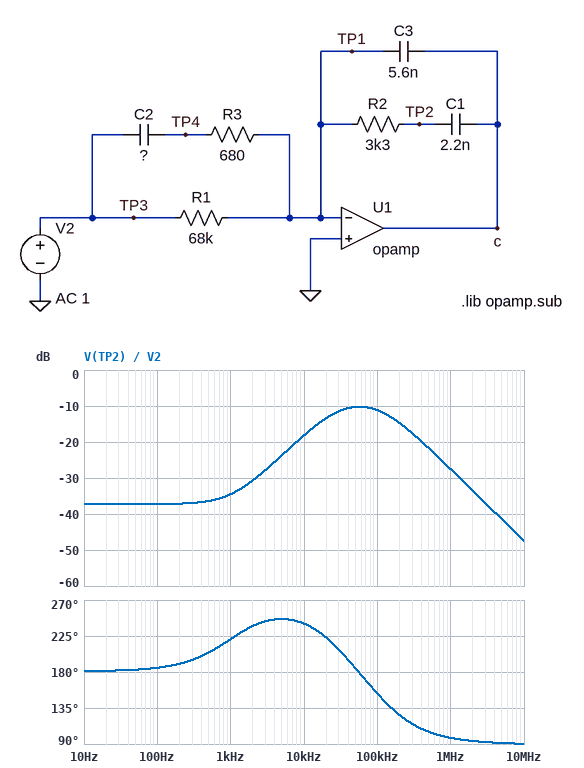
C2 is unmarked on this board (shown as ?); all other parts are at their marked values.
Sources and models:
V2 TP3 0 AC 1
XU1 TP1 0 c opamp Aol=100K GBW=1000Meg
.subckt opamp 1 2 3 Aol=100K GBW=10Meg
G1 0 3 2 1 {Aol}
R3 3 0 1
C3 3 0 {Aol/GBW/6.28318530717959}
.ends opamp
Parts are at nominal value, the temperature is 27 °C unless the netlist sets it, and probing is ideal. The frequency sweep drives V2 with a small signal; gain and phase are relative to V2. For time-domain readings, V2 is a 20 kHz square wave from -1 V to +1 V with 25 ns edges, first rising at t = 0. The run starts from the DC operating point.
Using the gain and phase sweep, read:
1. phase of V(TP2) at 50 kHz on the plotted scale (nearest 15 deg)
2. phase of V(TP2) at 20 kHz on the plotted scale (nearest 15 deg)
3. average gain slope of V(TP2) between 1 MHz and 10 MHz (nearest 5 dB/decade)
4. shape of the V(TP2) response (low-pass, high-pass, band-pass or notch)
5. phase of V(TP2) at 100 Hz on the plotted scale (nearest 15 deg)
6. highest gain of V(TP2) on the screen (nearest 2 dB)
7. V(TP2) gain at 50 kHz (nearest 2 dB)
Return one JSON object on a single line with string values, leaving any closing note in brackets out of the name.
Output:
{"phase of V(TP2) at 50 kHz on the plotted scale": "180 deg", "phase of V(TP2) at 20 kHz on the plotted scale": "225 deg", "average gain slope of V(TP2) between 1 MHz and 10 MHz": "-20 dB/decade", "shape of the V(TP2) response": "band-pass", "phase of V(TP2) at 100 Hz on the plotted scale": "180 deg", "highest gain of V(TP2) on the screen": "-10 dB", "V(TP2) gain at 50 kHz": "-10 dB"}
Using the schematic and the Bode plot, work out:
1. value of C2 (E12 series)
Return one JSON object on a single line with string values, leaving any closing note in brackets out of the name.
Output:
{"value of C2": "2.2 nF"}
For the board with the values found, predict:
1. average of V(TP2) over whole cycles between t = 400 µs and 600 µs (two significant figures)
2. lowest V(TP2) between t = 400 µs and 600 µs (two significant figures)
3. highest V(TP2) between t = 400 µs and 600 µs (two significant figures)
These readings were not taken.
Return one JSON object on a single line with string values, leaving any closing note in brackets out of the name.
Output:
{"average of V(TP2) over whole cycles between t = 400 µs and 600 µs": "-1.0 V", "lowest V(TP2) between t = 400 µs and 600 µs": "-1.5 V", "highest V(TP2) between t = 400 µs and 600 µs": "-550 mV"}
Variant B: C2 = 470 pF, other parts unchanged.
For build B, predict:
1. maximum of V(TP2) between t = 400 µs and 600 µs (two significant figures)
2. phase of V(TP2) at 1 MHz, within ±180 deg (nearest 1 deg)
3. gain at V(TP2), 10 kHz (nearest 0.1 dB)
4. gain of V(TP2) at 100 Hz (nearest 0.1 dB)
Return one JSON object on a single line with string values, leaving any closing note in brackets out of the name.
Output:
{"maximum of V(TP2) between t = 400 µs and 600 µs": "-880 mV", "phase of V(TP2) at 1 MHz, within ±180 deg": "118 deg", "gain at V(TP2), 10 kHz": "-30.6 dB", "gain of V(TP2) at 100 Hz": "-37.3 dB"}
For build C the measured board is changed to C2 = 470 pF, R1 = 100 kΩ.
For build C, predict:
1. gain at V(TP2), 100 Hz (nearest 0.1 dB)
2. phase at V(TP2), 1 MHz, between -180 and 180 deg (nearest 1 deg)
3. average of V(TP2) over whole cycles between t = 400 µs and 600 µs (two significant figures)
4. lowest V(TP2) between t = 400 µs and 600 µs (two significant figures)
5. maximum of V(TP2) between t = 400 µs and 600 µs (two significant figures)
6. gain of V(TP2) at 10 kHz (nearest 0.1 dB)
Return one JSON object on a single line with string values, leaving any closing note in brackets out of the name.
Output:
{"gain at V(TP2), 100 Hz": "-40.6 dB", "phase at V(TP2), 1 MHz, between -180 and 180 deg": "118 deg", "average of V(TP2) over whole cycles between t = 400 µs and 600 µs": "-1.0 V", "lowest V(TP2) between t = 400 µs and 600 µs": "-1.1 V", "maximum of V(TP2) between t = 400 µs and 600 µs": "-880 mV", "gain of V(TP2) at 10 kHz": "-31.1 dB"}
